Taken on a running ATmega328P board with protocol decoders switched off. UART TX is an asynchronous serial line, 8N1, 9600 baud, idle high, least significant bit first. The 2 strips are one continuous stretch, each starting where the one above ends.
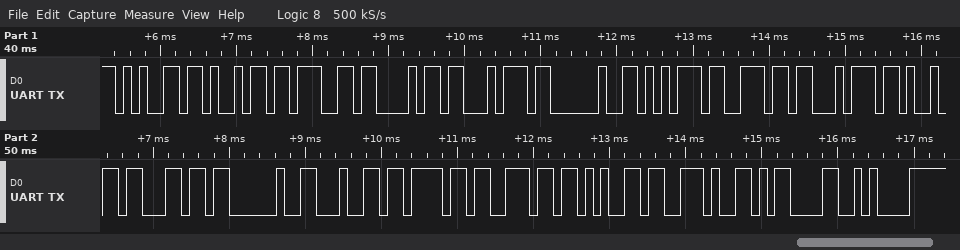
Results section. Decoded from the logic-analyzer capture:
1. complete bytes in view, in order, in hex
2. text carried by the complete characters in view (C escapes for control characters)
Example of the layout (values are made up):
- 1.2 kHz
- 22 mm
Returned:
- 65 69 67 68 74 20 75 6E 74 69 6C 20 64 6F 6E 65 2E 0D 0A
- "eight until done.\r\n"
